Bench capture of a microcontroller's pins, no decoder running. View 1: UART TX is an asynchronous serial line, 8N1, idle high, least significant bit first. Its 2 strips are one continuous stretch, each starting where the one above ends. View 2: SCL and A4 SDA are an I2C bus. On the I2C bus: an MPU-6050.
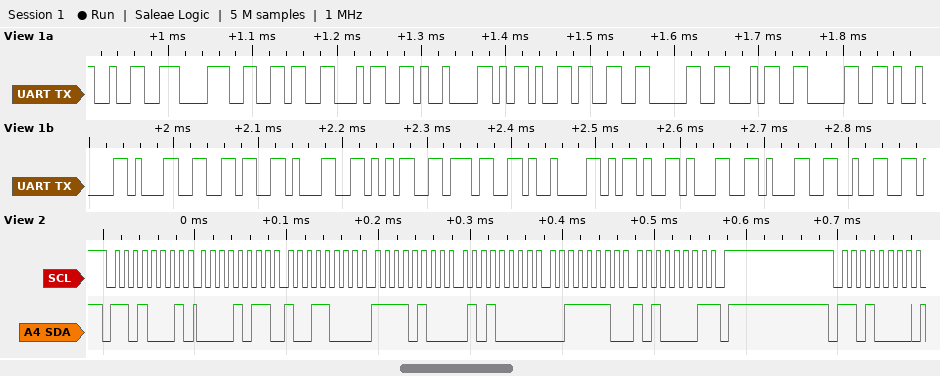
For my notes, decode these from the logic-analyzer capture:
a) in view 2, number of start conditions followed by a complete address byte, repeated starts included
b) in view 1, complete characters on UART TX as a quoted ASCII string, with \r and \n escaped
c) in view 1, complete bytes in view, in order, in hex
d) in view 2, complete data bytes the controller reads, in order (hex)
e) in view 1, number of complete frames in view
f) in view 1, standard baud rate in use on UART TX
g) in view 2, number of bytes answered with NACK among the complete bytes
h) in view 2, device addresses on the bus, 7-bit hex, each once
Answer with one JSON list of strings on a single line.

["2", "\"2864\\t-3040\\t16157\\t-112\"", "32 38 36 34 09 2D 33 30 34 30 09 31 36 31 35 37 09 2D 31 31 32", "0B 98 F4 50 3E A1", "21", "115200 baud", "1", "0x68"]
